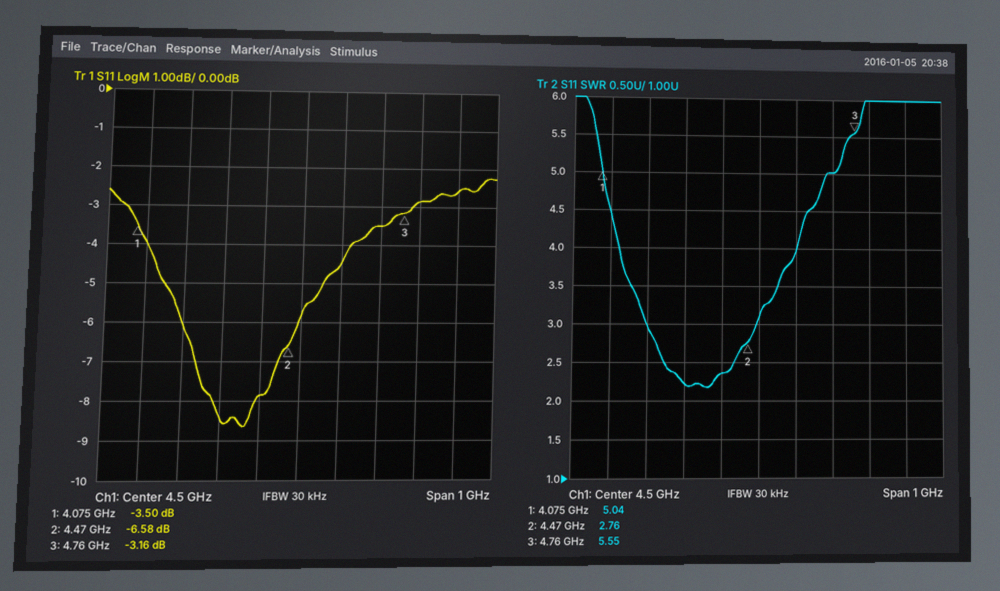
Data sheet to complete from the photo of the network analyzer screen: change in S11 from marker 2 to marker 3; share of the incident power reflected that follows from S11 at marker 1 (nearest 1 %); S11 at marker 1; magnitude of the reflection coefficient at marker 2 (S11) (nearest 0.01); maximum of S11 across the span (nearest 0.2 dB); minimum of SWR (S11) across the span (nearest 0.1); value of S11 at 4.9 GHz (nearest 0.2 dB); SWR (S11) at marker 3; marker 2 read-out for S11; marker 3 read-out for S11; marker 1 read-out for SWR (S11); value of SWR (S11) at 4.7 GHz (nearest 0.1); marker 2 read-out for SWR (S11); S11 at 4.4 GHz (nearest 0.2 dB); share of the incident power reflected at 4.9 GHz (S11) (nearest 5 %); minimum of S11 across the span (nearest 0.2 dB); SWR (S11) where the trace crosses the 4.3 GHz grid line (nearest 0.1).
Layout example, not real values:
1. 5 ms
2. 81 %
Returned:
1. 3.42 dB
2. 45 %
3. -3.50 dB
4. 0.47
5. -2.2 dB
6. 2.2
7. -2.6 dB
8. 5.55
9. -6.58 dB
10. -3.16 dB
11. 5.04
12. 5.0
13. 2.76
14. -7.8 dB
15. 55 %
16. -8.6 dB
17. 2.2
